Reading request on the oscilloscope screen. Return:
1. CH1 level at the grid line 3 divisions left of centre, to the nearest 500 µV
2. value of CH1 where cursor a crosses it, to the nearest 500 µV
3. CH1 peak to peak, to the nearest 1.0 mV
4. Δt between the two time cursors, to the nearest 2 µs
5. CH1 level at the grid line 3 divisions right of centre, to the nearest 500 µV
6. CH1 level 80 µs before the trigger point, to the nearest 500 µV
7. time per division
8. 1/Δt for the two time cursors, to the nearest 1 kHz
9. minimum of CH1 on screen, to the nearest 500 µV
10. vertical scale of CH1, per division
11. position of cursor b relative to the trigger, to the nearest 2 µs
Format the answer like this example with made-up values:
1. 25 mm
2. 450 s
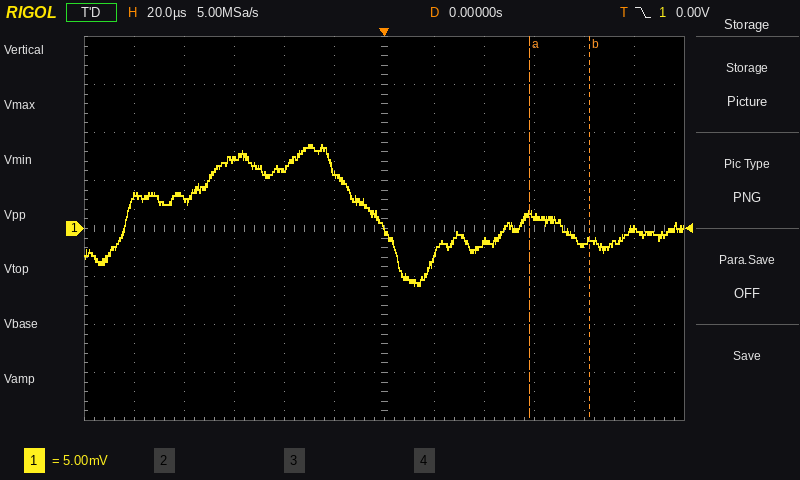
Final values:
1. 7.0 mV
2. 1.5 mV
3. 15.0 mV
4. 24 µs
5. 1.5 mV
6. 3.0 mV
7. 20 µs
8. 42 kHz
9. -6.0 mV
10. 5 mV
11. +82 µs
